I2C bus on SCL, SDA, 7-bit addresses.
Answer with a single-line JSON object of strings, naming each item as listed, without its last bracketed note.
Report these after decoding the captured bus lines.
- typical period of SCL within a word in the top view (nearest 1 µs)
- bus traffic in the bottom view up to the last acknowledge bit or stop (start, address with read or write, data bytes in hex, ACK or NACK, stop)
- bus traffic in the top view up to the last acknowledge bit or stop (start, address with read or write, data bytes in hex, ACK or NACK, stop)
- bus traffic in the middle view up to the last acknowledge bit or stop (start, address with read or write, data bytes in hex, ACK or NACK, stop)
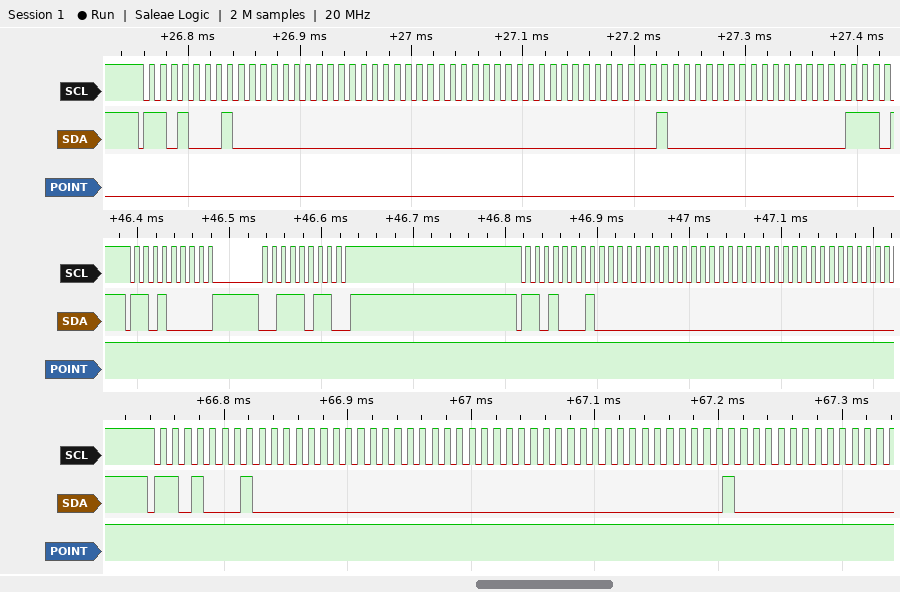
{"typical period of SCL within a word in the top view": "10 µs", "bus traffic in the bottom view up to the last acknowledge bit or stop": "start, address 68 read ACK, 00 ACK, 00 ACK, 00 ACK, 00 ACK, 40 ACK", "bus traffic in the top view up to the last acknowledge bit or stop": "start, address 68 read ACK, 00 ACK, 00 ACK, 00 ACK, 00 ACK, 40 ACK, 00 ACK", "bus traffic in the middle view up to the last acknowledge bit or stop": "start, address 68 write ACK, 3B ACK, stop, start, address 68 read ACK, 00 ACK, 00 ACK, 00 ACK"}
